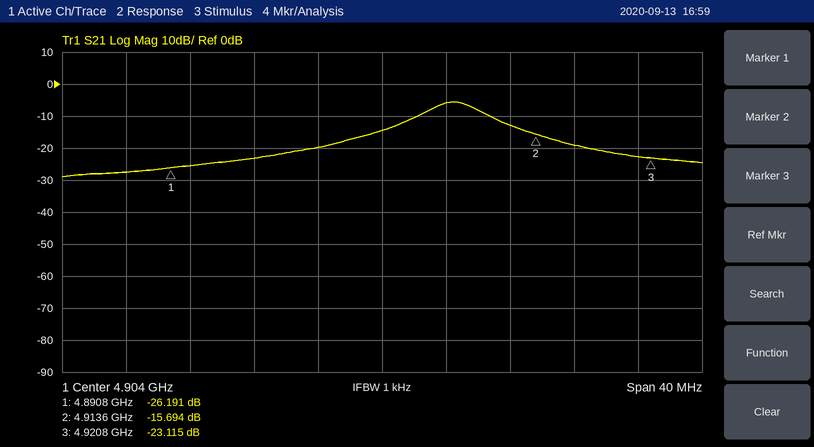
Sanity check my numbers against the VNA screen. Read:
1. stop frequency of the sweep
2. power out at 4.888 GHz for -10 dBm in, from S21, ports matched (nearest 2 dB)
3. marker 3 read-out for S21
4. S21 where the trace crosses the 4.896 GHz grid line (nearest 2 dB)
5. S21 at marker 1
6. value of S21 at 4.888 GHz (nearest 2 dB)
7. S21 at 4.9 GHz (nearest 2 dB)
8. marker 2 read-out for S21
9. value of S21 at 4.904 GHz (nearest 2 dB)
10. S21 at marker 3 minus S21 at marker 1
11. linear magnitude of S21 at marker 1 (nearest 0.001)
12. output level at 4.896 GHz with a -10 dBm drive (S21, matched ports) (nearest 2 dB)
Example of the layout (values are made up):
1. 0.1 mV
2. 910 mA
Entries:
1. 4.924 GHz
2. -38 dBm
3. -23.115 dB
4. -24 dB
5. -26.191 dB
6. -28 dB
7. -20 dB
8. -15.694 dB
9. -14 dB
10. 3.076 dB
11. 0.049
12. -34 dBm
